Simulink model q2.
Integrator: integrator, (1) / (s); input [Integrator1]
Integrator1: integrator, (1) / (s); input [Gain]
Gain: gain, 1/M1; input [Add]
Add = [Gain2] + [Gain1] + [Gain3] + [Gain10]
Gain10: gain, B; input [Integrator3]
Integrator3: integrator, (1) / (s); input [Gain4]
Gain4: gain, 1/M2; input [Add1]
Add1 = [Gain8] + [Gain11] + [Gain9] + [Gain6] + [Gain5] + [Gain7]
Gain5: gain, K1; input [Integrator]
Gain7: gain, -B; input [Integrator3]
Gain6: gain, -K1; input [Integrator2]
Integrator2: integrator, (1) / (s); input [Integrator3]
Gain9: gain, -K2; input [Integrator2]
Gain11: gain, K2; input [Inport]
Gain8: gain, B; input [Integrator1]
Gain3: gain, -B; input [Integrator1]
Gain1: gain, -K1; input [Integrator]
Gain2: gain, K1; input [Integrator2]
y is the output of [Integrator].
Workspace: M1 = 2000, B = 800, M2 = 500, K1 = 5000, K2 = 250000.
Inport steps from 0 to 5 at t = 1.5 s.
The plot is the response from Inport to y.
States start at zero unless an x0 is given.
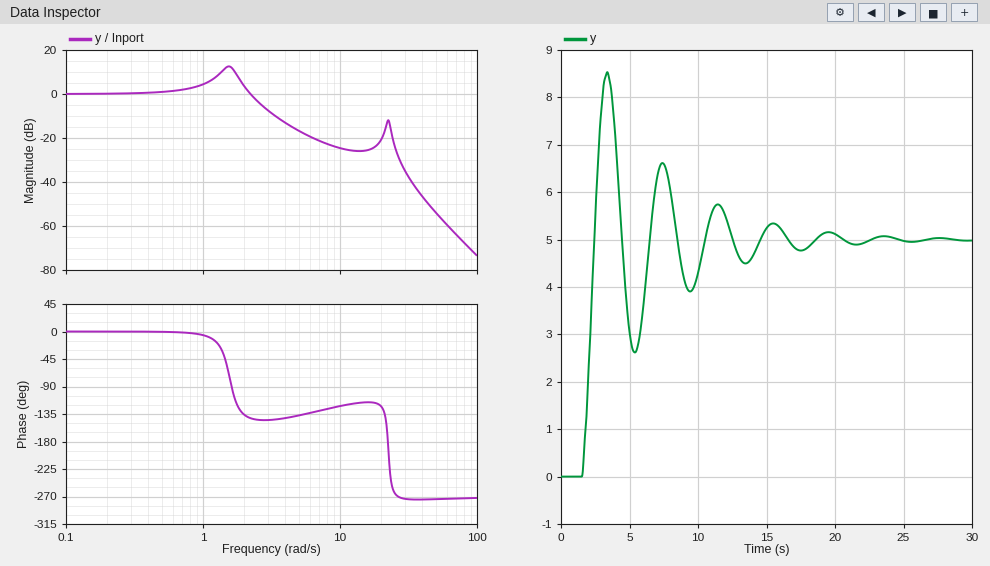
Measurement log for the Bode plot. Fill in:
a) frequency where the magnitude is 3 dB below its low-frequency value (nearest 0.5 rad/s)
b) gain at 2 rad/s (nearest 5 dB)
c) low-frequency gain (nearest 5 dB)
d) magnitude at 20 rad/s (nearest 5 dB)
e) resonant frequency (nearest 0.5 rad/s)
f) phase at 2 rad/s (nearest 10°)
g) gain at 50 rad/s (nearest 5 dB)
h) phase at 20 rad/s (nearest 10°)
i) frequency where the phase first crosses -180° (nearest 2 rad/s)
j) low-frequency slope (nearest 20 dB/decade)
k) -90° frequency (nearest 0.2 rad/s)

2.5 rad/s
5 dB
0 dB
-20 dB
1.5 rad/s
-140°
-55 dB
-120°
22 rad/s
0 dB/decade
1.6 rad/s
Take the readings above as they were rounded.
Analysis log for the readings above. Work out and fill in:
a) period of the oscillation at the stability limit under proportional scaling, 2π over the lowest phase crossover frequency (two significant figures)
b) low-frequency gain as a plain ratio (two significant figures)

0.29 s
1.0
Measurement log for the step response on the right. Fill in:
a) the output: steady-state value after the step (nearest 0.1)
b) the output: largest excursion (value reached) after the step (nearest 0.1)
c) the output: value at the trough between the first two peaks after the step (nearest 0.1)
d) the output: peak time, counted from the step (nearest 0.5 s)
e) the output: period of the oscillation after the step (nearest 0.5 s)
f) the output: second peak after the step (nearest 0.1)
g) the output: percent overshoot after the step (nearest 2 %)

5.0
8.5
2.6
2.0 s
4.0 s
6.6
70 %
